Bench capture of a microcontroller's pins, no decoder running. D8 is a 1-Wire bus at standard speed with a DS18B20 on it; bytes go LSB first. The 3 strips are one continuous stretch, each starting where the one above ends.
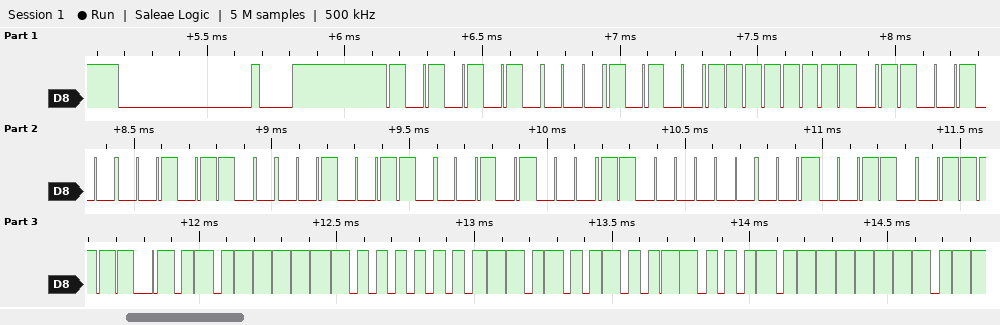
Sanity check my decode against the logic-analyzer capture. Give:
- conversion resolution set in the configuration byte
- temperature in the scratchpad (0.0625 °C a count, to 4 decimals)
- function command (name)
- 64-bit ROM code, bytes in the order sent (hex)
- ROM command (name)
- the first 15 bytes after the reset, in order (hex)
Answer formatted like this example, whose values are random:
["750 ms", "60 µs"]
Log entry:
["12 bits", "31.6250 °C", "Read Scratchpad", "28 FF 26 34 64 14 03 64", "Match ROM", "55 28 FF 26 34 64 14 03 64 BE FA 01 4B 46 7F"]
